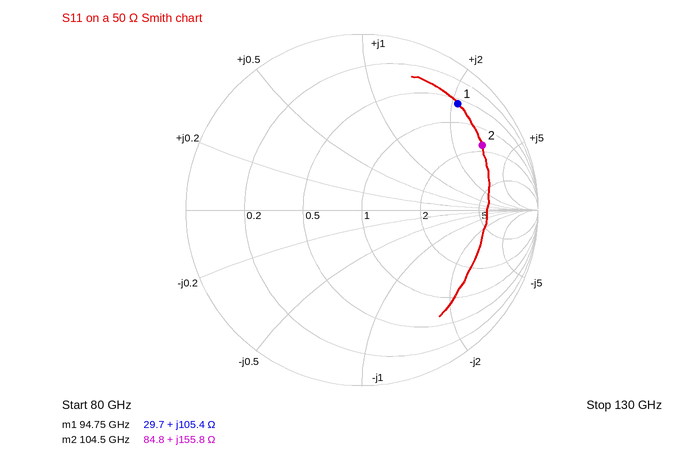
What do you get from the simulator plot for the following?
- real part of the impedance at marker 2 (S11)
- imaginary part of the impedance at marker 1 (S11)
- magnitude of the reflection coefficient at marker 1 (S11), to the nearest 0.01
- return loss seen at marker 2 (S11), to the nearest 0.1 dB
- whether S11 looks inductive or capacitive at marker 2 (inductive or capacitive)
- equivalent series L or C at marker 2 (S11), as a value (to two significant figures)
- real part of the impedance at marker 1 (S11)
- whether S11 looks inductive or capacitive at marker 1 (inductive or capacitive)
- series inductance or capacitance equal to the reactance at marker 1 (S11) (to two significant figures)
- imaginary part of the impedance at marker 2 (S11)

84.8 Ω
+105.4 Ω
0.81
2.2 dB
inductive
240 pH
29.7 Ω
inductive
180 pH
+155.8 Ω
